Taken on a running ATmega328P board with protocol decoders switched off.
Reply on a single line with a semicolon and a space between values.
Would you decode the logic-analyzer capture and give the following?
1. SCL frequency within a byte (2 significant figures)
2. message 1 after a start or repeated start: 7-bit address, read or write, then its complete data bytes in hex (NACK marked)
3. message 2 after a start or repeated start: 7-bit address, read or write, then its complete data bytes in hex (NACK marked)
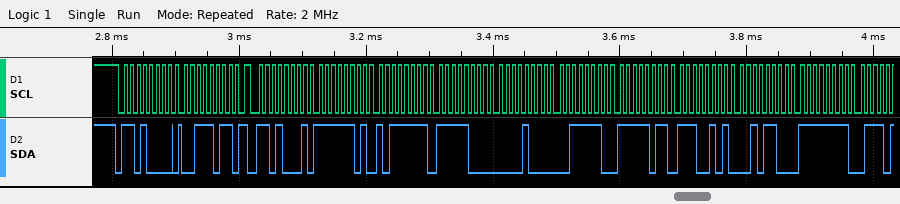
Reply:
100 kHz; 0x68 write: 3B; 0x68 read: FD BF F8 08 3E FB E5 2C FF
